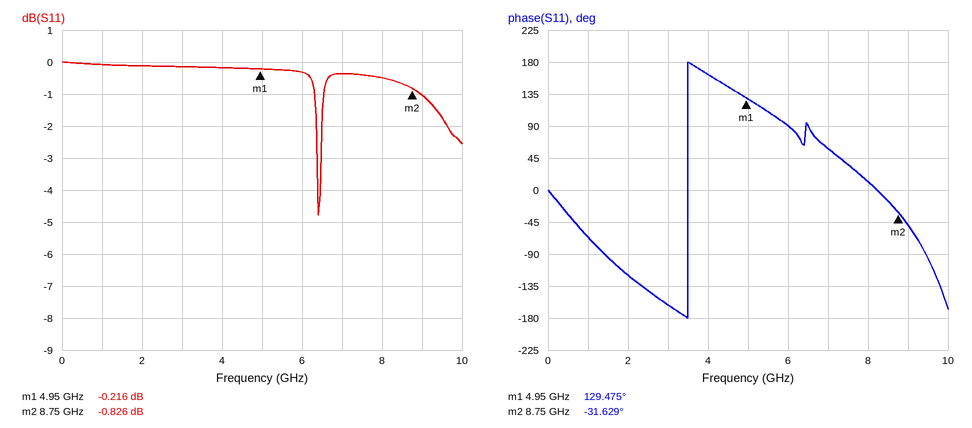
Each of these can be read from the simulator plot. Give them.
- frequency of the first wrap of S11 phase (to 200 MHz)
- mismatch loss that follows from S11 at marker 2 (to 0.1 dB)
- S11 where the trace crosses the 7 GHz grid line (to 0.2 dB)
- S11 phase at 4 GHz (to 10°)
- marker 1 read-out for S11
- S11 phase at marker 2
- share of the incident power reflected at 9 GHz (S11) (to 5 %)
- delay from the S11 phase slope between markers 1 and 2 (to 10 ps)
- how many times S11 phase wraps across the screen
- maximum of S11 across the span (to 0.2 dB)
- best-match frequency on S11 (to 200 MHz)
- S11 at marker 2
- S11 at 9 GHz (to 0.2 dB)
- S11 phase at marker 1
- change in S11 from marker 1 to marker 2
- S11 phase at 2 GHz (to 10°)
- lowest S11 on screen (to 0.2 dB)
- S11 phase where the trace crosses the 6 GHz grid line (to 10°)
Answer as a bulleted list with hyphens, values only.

- 3.4 GHz
- 7.6 dB
- -0.4 dB
- 160°
- -0.216 dB
- -31.629°
- 80 %
- 120 ps
- 1
- 0.0 dB
- 6.4 GHz
- -0.826 dB
- -1.0 dB
- 129.475°
- -0.610 dB
- -120°
- -4.8 dB
- 90°
